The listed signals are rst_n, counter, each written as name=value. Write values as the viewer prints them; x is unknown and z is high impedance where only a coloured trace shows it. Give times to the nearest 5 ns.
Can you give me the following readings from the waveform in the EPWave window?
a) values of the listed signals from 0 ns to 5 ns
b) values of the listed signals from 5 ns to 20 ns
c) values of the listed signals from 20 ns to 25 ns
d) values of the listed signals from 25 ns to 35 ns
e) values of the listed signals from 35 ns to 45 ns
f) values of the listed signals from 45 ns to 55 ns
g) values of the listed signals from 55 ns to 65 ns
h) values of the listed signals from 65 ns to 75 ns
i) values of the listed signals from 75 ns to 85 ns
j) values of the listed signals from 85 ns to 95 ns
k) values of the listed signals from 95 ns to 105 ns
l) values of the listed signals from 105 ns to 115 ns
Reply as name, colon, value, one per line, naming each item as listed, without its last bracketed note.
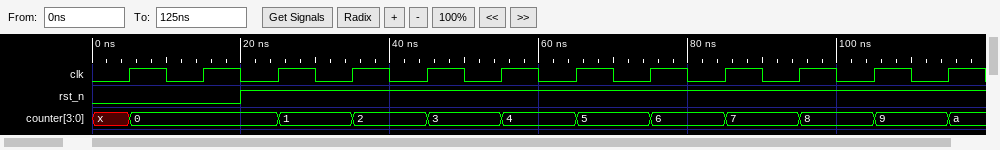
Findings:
values of the listed signals from 0 ns to 5 ns: rst_n=0, counter=x
values of the listed signals from 5 ns to 20 ns: rst_n=0, counter=0
values of the listed signals from 20 ns to 25 ns: rst_n=1, counter=0
values of the listed signals from 25 ns to 35 ns: rst_n=1, counter=1
values of the listed signals from 35 ns to 45 ns: rst_n=1, counter=2
values of the listed signals from 45 ns to 55 ns: rst_n=1, counter=3
values of the listed signals from 55 ns to 65 ns: rst_n=1, counter=4
values of the listed signals from 65 ns to 75 ns: rst_n=1, counter=5
values of the listed signals from 75 ns to 85 ns: rst_n=1, counter=6
values of the listed signals from 85 ns to 95 ns: rst_n=1, counter=7
values of the listed signals from 95 ns to 105 ns: rst_n=1, counter=8
values of the listed signals from 105 ns to 115 ns: rst_n=1, counter=9
